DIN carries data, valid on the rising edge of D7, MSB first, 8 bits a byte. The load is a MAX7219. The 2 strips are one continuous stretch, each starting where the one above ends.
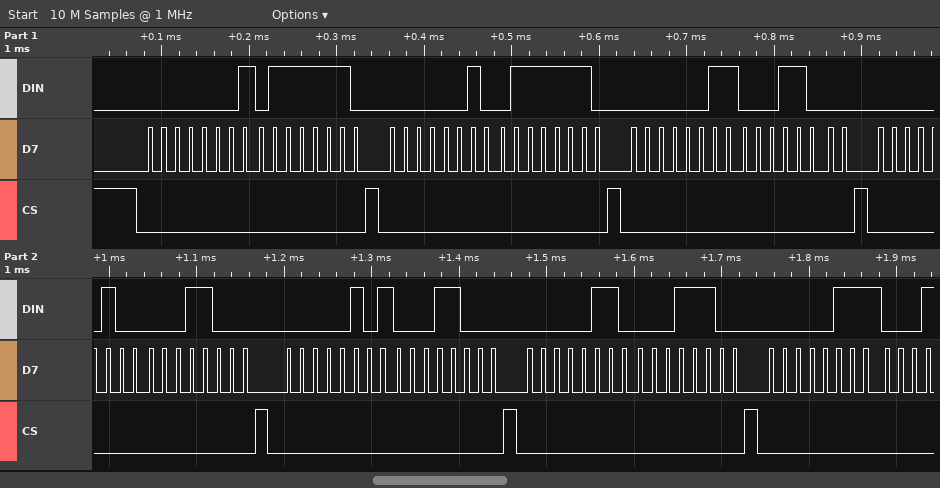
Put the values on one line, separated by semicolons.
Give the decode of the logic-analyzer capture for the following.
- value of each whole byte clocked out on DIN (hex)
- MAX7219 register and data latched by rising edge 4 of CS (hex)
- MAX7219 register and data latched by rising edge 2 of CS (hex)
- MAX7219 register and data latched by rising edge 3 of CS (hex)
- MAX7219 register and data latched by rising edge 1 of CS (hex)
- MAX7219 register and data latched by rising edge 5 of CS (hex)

01 7E 02 7E 03 18 04 18 05 18 06 1C 07; register 0x4, data 0x18; register 0x2, data 0x7E; register 0x3, data 0x18; register 0x1, data 0x7E; register 0x5, data 0x18
